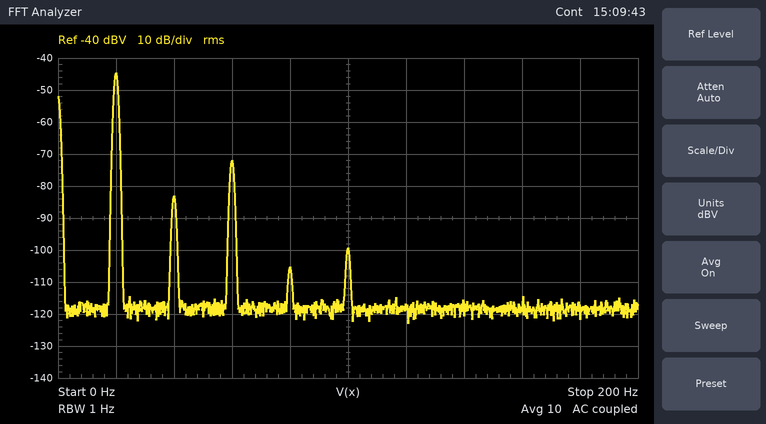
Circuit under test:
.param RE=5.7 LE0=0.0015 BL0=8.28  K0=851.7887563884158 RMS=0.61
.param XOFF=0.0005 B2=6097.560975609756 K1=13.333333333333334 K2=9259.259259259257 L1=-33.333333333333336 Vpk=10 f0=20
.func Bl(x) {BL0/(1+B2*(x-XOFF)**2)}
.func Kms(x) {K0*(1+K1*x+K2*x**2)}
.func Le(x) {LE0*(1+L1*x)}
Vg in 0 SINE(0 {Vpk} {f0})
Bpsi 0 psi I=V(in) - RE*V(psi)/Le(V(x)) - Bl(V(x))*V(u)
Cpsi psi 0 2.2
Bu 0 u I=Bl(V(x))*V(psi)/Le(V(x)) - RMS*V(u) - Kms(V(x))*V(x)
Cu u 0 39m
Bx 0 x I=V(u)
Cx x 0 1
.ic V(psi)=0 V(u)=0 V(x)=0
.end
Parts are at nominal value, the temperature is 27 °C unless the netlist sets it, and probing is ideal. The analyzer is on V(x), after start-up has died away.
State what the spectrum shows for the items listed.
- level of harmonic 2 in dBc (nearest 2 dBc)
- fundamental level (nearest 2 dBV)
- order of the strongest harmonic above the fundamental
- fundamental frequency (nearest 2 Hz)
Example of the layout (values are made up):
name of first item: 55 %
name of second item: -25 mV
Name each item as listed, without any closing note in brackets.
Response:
level of harmonic 2 in dBc: -38 dBc
fundamental level: -44 dBV
order of the strongest harmonic above the fundamental: 3
fundamental frequency: 20 Hz
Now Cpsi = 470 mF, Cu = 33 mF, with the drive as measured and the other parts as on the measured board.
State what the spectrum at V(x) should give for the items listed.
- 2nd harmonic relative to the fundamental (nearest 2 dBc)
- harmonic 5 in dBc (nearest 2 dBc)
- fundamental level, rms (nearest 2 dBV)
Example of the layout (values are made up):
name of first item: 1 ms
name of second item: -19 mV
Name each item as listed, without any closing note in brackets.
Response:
2nd harmonic relative to the fundamental: -36 dBc
harmonic 5 in dBc: -52 dBc
fundamental level, rms: -44 dBV
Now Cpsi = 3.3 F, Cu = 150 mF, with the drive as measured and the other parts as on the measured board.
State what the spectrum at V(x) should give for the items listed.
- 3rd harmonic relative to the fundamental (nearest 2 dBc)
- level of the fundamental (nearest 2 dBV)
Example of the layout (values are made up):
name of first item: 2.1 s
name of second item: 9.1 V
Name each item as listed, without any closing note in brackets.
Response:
3rd harmonic relative to the fundamental: -50 dBc
level of the fundamental: -46 dBV
